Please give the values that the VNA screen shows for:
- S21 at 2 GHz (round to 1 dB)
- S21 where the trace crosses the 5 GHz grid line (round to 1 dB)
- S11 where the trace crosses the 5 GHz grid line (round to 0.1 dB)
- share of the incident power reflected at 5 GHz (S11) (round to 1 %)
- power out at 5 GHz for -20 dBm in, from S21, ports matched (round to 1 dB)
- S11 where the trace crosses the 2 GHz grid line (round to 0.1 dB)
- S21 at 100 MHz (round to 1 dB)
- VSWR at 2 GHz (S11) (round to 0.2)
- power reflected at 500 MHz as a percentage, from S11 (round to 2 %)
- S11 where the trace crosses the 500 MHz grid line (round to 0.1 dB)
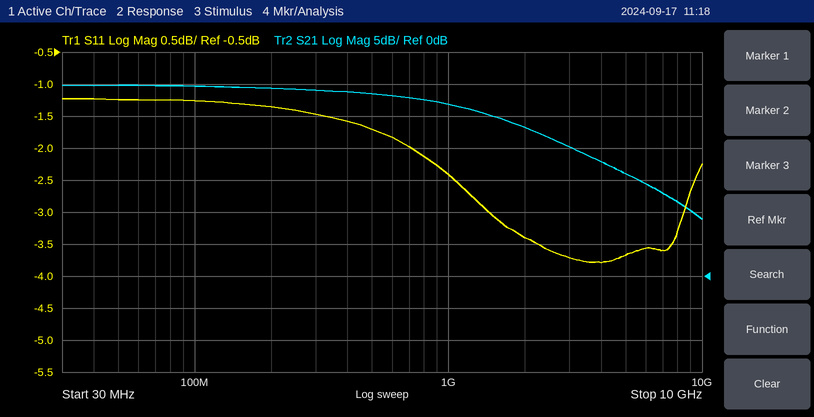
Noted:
23 dB
16 dB
-3.7 dB
43 %
-4 dBm
-3.4 dB
30 dB
5.2
68 %
-1.7 dB
